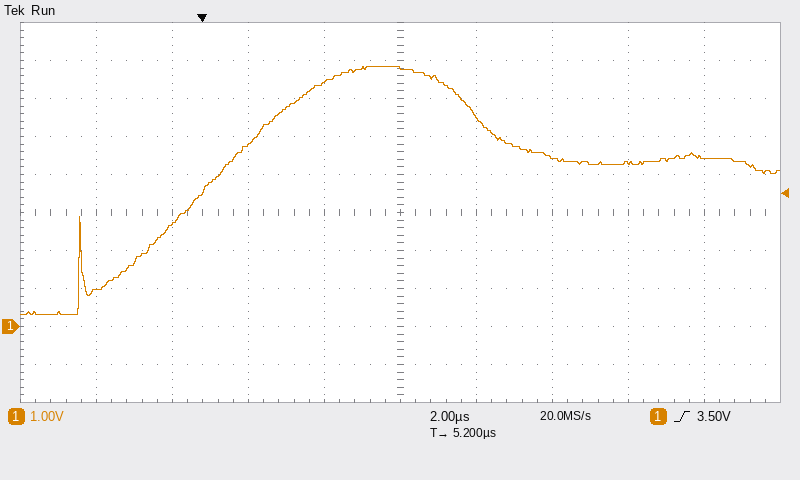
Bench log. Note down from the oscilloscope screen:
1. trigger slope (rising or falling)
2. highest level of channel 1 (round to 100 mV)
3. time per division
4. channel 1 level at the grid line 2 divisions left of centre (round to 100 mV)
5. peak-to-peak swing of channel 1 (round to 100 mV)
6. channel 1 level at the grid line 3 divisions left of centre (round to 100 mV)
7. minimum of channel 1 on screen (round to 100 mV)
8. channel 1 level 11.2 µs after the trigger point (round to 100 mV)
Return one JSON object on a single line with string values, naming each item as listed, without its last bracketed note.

{"trigger slope": "rising", "highest level of channel 1": "6.8 V", "time per division": "2 µs", "channel 1 level at the grid line 2 divisions left of centre": "4.8 V", "peak-to-peak swing of channel 1": "6.5 V", "channel 1 level at the grid line 3 divisions left of centre": "2.7 V", "minimum of channel 1 on screen": "300 mV", "channel 1 level 11.2 µs after the trigger point": "4.3 V"}
